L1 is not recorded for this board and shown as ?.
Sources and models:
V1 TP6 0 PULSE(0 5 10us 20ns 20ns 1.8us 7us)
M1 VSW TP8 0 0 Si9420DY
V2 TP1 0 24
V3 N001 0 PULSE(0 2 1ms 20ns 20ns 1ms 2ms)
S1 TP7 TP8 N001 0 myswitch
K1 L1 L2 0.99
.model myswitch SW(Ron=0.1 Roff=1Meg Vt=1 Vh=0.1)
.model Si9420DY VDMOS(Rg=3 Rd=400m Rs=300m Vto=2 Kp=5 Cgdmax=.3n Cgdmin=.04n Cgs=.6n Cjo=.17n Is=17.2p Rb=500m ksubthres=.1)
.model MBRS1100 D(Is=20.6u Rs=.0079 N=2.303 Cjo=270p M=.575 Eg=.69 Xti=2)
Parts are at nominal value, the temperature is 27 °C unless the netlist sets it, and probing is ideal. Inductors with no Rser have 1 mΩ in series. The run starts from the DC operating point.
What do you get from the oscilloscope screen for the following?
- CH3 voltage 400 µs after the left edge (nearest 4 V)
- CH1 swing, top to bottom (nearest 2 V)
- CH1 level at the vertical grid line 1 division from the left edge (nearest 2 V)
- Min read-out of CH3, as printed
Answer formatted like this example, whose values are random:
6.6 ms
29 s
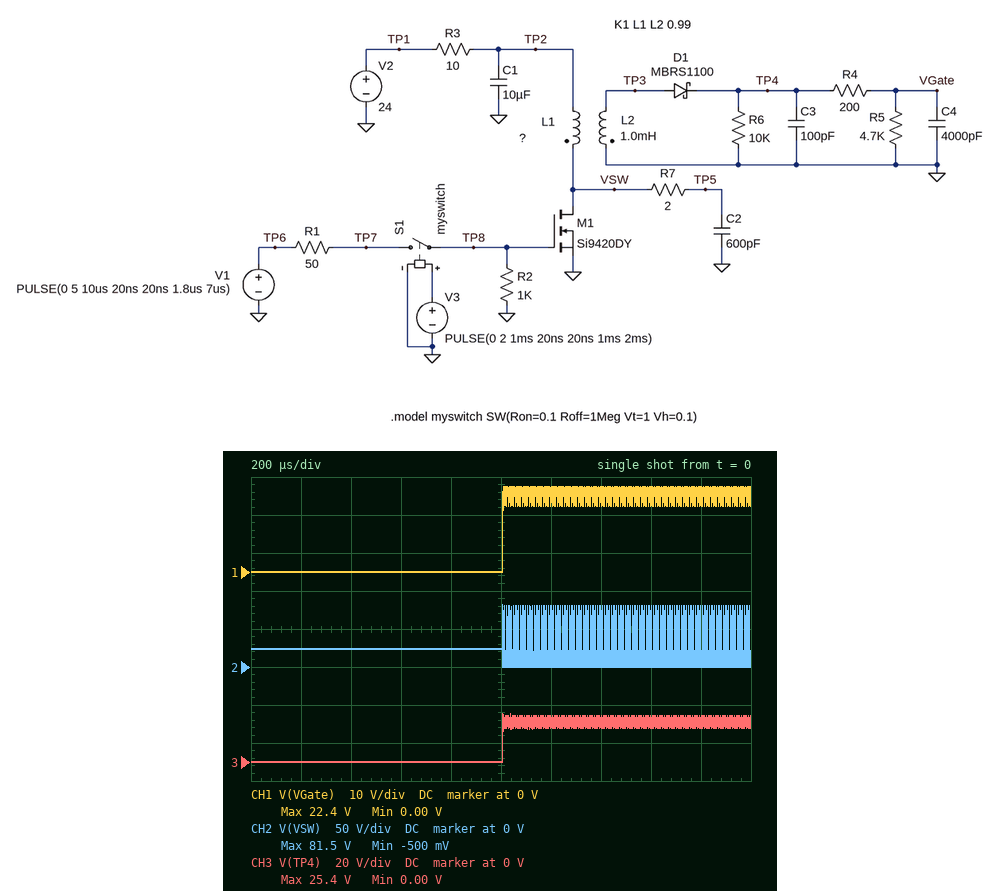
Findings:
0 V
22 V
0 V
0.00 V
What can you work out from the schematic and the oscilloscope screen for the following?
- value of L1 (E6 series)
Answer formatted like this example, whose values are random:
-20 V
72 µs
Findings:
1 mH
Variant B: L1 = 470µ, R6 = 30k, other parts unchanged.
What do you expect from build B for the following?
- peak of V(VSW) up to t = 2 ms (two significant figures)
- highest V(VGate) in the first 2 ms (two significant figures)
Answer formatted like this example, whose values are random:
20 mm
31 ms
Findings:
130 V
33 V
